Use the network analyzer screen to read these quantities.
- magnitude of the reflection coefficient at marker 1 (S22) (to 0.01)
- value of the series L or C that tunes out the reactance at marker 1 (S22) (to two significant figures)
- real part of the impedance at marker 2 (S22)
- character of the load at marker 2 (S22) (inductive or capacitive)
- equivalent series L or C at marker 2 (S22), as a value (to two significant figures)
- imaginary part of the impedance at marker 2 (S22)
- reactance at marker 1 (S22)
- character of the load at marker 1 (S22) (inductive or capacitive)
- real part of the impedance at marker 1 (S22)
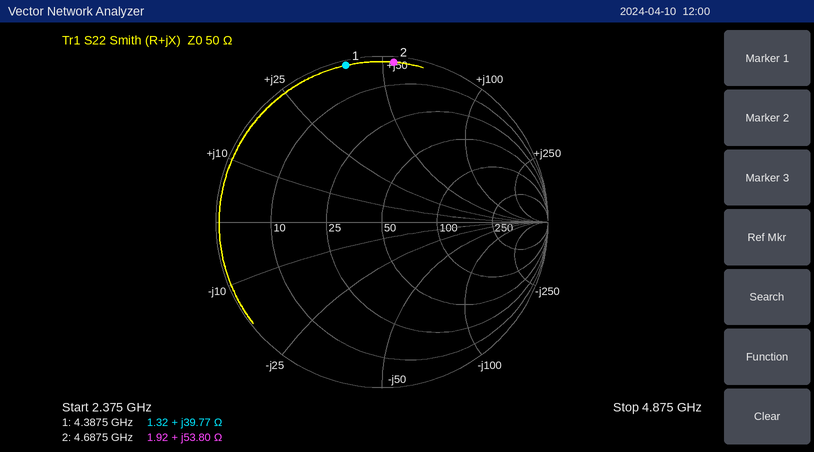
0.97
910 fF
1.92 Ω
inductive
1.8 nH
+53.80 Ω
+39.77 Ω
inductive
1.32 Ω
